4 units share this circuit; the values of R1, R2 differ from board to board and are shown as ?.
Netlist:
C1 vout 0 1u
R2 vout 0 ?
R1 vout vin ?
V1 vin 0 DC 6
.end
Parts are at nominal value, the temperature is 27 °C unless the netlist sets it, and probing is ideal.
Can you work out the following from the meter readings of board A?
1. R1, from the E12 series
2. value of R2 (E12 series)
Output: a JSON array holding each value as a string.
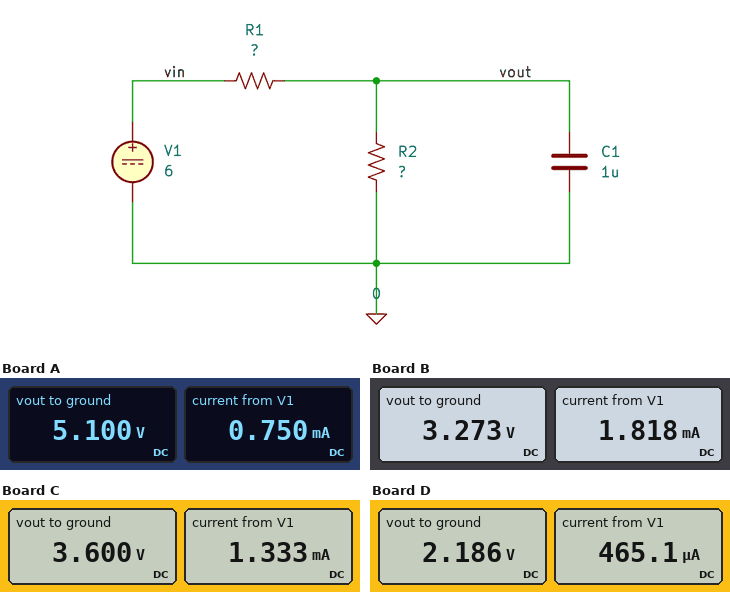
["1.2 kΩ", "6.8 kΩ"]
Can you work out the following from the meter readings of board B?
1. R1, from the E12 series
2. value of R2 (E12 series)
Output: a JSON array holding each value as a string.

["1.5 kΩ", "1.8 kΩ"]
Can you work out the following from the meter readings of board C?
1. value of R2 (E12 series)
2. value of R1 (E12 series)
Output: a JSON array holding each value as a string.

["2.7 kΩ", "1.8 kΩ"]
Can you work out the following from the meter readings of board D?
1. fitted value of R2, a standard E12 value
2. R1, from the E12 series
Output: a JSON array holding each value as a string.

["4.7 kΩ", "8.2 kΩ"]
